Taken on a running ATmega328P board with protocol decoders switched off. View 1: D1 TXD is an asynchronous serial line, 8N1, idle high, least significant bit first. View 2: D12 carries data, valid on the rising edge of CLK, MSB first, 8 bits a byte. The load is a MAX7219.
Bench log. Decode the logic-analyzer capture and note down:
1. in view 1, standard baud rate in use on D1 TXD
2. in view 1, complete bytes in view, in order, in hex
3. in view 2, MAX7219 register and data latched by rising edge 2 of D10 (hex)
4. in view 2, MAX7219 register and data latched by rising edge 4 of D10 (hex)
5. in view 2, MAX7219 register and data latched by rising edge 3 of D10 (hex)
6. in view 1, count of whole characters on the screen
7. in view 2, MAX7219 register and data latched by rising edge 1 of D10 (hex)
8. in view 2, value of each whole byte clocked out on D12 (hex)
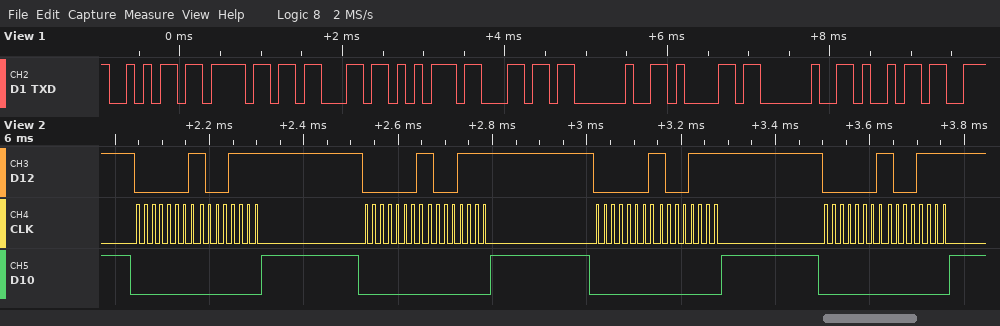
9600 baud
6A 6F 63 75 6C 20 61 20 69
register 0x1, data 0x8F
register 0x1, data 0x8F
register 0x1, data 0x8F
9
register 0x1, data 0x8F
01 8F 01 8F 01 8F 01 8F
